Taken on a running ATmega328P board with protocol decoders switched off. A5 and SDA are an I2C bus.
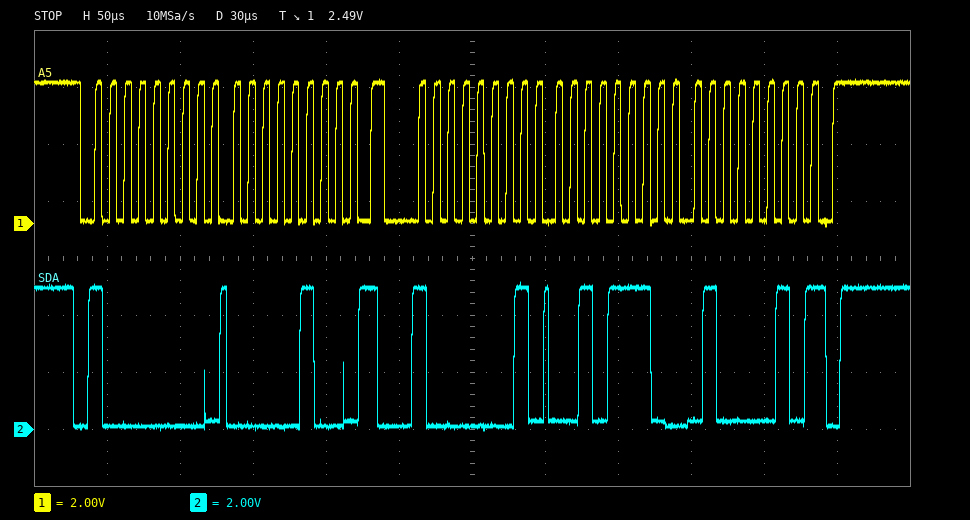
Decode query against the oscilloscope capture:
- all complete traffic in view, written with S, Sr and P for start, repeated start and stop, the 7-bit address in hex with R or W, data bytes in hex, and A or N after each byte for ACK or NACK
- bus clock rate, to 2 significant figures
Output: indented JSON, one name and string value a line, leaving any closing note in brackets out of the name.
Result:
{
  "all complete traffic in view, written with S, Sr and P for start, repeated start and stop, the 7-bit address in hex with R or W, data bytes in hex, and A or N after each byte for ACK or NACK": "S 40W A 04 A Sr 40R A 2E A 42 N P",
  "bus clock rate, to 2 significant figures": "100 kHz"
}
